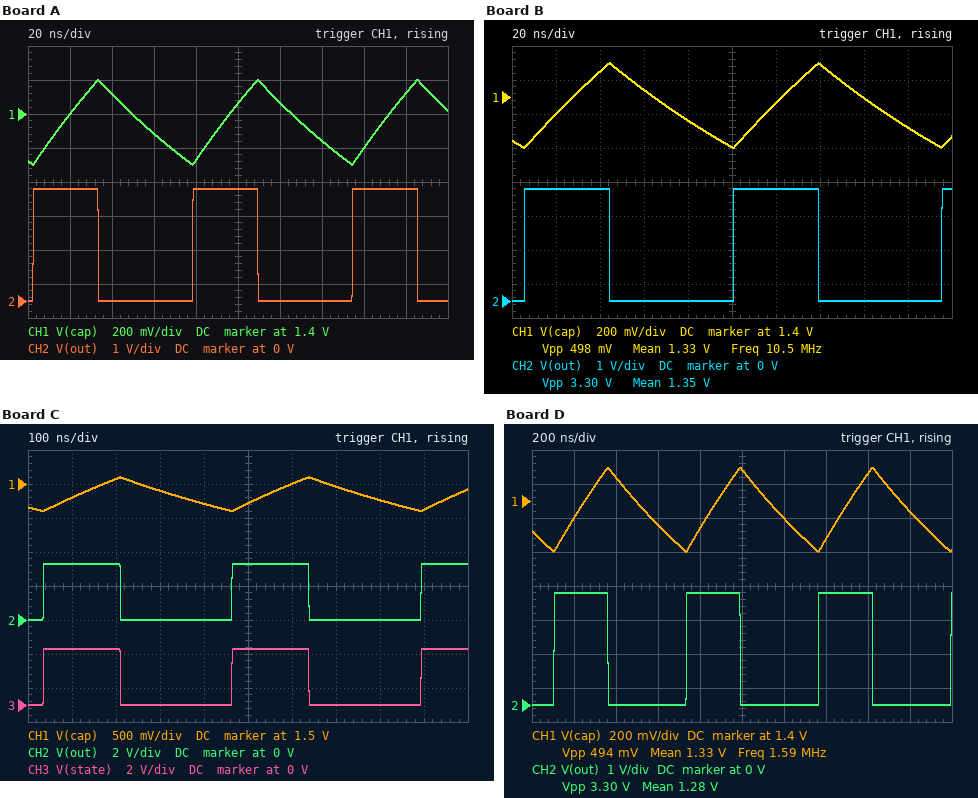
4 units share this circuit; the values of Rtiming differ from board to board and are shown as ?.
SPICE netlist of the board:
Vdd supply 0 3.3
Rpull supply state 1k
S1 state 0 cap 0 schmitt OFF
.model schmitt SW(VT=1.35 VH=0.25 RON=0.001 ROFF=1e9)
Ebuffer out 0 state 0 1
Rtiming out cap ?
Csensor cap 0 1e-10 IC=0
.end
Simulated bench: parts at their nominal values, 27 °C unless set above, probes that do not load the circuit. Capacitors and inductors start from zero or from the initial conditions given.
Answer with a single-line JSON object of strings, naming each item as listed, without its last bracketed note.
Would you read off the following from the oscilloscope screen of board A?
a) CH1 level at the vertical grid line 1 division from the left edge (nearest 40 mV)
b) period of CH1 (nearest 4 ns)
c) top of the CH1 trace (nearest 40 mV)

{"CH1 level at the vertical grid line 1 division from the left edge": "1.40 V", "period of CH1": "76 ns", "top of the CH1 trace": "1.60 V"}
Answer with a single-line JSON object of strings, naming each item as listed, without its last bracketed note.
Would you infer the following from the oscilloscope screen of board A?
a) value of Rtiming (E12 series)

{"value of Rtiming": "1.2 kΩ"}
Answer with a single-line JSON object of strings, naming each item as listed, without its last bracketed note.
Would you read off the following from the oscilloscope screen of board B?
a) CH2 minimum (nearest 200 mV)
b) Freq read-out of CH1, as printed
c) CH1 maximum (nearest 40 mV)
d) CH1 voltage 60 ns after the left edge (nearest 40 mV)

{"CH2 minimum": "0 V", "Freq read-out of CH1, as printed": "10.5 MHz", "CH1 maximum": "1.60 V", "CH1 voltage 60 ns after the left edge": "1.44 V"}
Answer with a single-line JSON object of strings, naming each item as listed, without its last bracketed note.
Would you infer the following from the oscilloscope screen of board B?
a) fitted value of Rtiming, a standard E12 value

{"fitted value of Rtiming, a standard E12 value": "1.5 kΩ"}
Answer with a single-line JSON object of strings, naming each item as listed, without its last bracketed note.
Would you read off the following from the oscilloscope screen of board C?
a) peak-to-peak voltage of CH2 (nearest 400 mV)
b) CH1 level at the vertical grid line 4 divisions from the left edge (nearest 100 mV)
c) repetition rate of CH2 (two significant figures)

{"peak-to-peak voltage of CH2": "3.2 V", "CH1 level at the vertical grid line 4 divisions from the left edge": "1.2 V", "repetition rate of CH2": "2.3 MHz"}
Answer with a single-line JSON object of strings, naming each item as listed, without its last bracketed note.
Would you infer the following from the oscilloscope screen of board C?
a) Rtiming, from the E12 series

{"Rtiming, from the E12 series": "6.8 kΩ"}
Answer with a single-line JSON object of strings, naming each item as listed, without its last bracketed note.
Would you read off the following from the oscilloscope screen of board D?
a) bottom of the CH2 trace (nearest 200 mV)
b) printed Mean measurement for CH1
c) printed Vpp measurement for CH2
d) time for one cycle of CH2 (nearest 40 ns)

{"bottom of the CH2 trace": "0 V", "printed Mean measurement for CH1": "1.33 V", "printed Vpp measurement for CH2": "3.30 V", "time for one cycle of CH2": "640 ns"}
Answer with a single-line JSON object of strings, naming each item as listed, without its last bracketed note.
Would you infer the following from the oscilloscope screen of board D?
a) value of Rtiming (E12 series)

{"value of Rtiming": "10 kΩ"}
